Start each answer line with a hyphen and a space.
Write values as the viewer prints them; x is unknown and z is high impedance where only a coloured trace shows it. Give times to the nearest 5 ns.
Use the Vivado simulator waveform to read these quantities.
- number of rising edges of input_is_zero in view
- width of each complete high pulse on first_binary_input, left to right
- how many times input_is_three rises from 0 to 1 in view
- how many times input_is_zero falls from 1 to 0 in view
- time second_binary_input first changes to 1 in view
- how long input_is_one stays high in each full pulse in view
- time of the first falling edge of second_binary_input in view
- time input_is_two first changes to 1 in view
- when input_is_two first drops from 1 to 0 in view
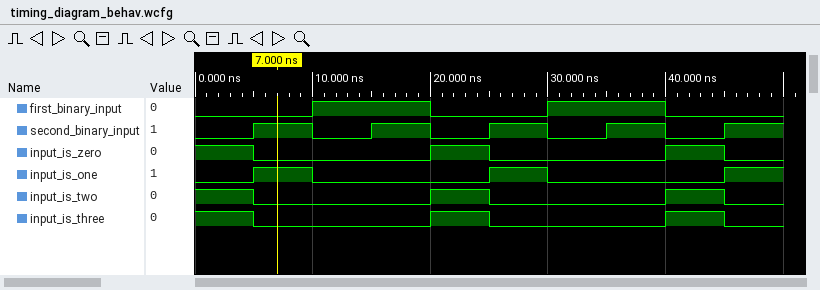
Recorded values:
- 2
- 10 ns, 10 ns
- 2
- 3
- 5 ns
- 5 ns, 5 ns
- 10 ns
- 20 ns
- 5 ns
